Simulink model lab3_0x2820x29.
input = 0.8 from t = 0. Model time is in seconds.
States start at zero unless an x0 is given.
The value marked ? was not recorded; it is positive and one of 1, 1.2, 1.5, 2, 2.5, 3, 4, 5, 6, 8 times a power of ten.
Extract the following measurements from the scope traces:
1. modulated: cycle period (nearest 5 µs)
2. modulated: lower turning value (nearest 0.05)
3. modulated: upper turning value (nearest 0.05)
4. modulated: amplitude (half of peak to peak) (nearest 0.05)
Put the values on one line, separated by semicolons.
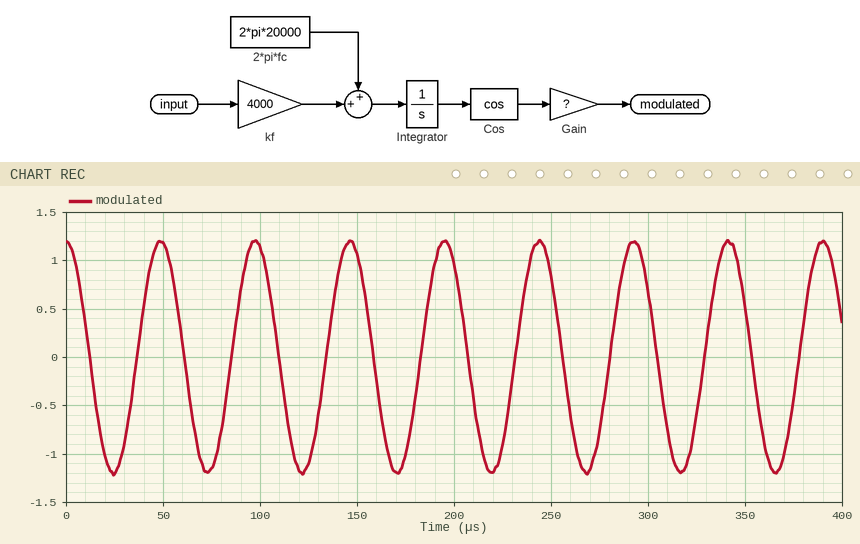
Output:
50 µs; -1.20; 1.20; 1.20
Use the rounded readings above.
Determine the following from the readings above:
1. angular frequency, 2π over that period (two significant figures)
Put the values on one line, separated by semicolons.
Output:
0.13 rad/µs
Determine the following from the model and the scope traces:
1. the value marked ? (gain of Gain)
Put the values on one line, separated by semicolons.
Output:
1.2
